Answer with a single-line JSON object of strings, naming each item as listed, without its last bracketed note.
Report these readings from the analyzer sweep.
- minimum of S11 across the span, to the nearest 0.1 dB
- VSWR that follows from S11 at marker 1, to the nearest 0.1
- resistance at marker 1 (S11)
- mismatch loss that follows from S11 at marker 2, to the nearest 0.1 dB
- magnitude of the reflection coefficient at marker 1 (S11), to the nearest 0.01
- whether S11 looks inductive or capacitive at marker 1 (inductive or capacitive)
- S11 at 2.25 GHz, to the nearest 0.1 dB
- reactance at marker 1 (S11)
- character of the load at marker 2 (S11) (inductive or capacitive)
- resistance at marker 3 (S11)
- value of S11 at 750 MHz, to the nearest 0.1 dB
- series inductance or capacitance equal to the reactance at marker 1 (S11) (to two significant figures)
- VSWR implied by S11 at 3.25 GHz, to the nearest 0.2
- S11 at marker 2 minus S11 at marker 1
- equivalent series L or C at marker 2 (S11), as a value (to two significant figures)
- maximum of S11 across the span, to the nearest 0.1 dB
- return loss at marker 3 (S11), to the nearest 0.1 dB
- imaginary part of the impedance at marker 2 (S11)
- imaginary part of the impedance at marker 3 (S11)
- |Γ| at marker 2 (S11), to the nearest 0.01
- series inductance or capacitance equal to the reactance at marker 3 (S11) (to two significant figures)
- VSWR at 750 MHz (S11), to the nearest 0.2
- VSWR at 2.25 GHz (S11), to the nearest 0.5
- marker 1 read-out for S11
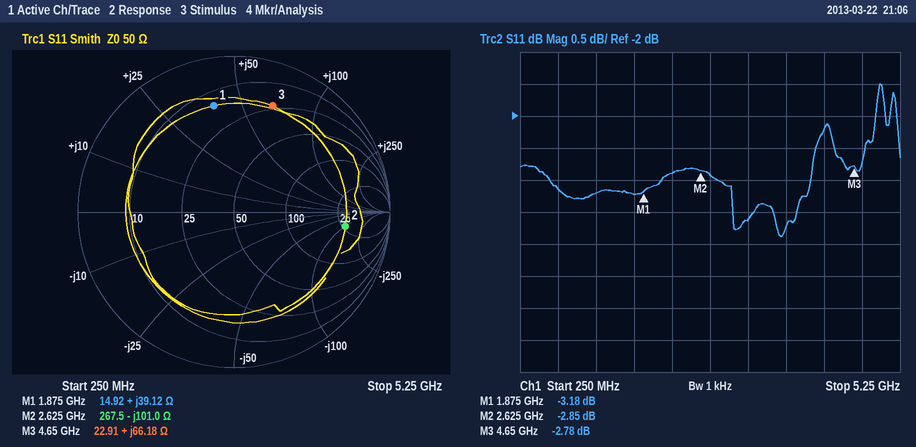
{"minimum of S11 across the span, to the nearest 0.1 dB": "-3.9 dB", "VSWR that follows from S11 at marker 1, to the nearest 0.1": "5.5", "resistance at marker 1": "14.92 Ω", "mismatch loss that follows from S11 at marker 2, to the nearest 0.1 dB": "3.2 dB", "magnitude of the reflection coefficient at marker 1 (S11), to the nearest 0.01": "0.69", "whether S11 looks inductive or capacitive at marker 1": "inductive", "S11 at 2.25 GHz, to the nearest 0.1 dB": "-2.9 dB", "reactance at marker 1": "+39.12 Ω", "character of the load at marker 2 (S11)": "capacitive", "resistance at marker 3": "22.91 Ω", "value of S11 at 750 MHz, to the nearest 0.1 dB": "-3.1 dB", "series inductance or capacitance equal to the reactance at marker 1 (S11)": "3.3 nH", "VSWR implied by S11 at 3.25 GHz, to the nearest 0.2": "4.8", "S11 at marker 2 minus S11 at marker 1": "0.33 dB", "equivalent series L or C at marker 2 (S11), as a value": "600 fF", "maximum of S11 across the span, to the nearest 0.1 dB": "-1.5 dB", "return loss at marker 3 (S11), to the nearest 0.1 dB": "2.8 dB", "imaginary part of the impedance at marker 2": "-101.0 Ω", "imaginary part of the impedance at marker 3": "+66.18 Ω", "|Γ| at marker 2 (S11), to the nearest 0.01": "0.72", "series inductance or capacitance equal to the reactance at marker 3 (S11)": "2.3 nH", "VSWR at 750 MHz (S11), to the nearest 0.2": "5.6", "VSWR at 2.25 GHz (S11), to the nearest 0.5": "6.0", "marker 1 read-out for S11": "-3.18 dB"}
